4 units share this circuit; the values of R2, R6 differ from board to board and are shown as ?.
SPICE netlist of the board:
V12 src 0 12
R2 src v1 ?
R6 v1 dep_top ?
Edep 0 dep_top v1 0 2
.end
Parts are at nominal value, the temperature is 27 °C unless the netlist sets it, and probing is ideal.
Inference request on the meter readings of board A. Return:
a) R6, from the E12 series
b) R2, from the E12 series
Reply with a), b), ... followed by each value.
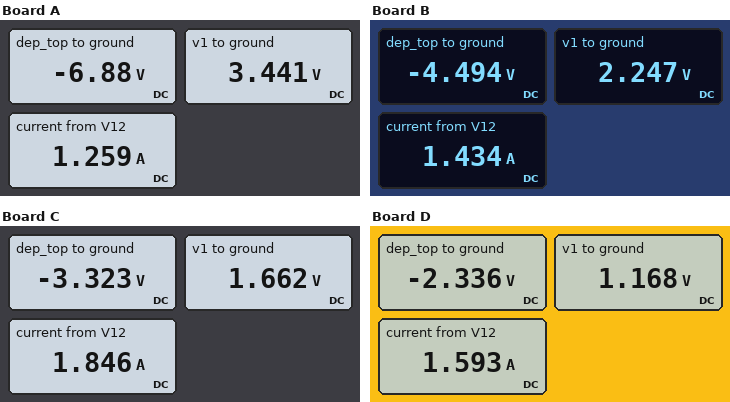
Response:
a) 8.2 Ω
b) 6.8 Ω
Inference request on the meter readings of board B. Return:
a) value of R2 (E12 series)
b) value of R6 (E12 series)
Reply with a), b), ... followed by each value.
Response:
a) 6.8 Ω
b) 4.7 Ω
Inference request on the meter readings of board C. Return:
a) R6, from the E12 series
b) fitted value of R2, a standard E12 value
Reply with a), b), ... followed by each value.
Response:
a) 2.7 Ω
b) 5.6 Ω
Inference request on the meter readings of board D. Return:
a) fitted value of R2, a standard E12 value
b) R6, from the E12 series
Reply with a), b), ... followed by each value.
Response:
a) 6.8 Ω
b) 2.2 Ω
